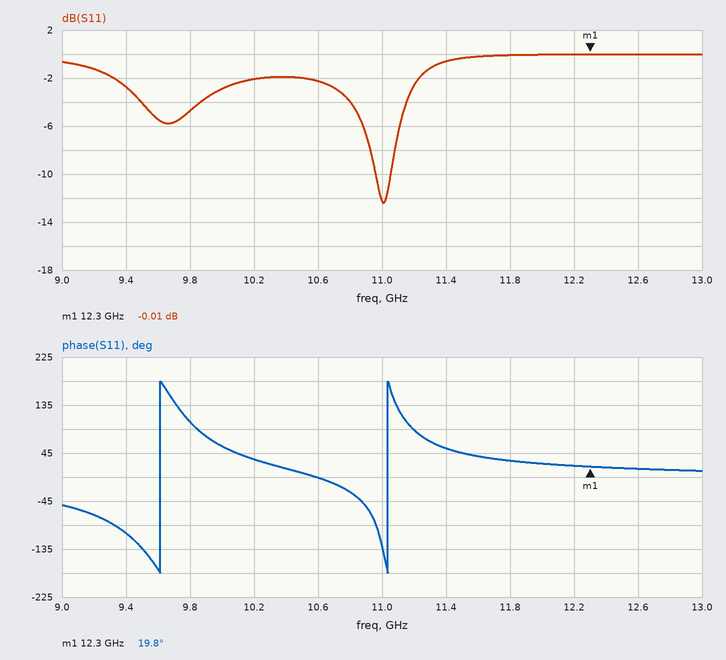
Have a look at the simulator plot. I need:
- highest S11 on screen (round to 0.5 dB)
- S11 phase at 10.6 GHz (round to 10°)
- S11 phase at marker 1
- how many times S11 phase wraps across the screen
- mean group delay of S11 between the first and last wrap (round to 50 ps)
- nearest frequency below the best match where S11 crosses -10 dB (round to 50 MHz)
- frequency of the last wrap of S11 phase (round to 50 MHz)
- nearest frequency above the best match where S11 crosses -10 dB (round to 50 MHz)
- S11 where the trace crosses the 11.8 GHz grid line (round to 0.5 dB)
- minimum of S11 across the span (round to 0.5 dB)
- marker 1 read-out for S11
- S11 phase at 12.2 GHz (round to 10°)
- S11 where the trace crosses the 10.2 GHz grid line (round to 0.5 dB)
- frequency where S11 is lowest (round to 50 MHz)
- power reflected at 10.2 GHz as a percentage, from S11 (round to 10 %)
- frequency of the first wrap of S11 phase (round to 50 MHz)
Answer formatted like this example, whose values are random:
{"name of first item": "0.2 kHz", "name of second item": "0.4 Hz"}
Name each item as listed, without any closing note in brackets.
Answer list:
{"highest S11 on screen": "0.0 dB", "S11 phase at 10.6 GHz": "0°", "S11 phase at marker 1": "19.8°", "how many times S11 phase wraps across the screen": "2", "mean group delay of S11 between the first and last wrap": "700 ps", "nearest frequency below the best match where S11 crosses -10 dB": "10.95 GHz", "frequency of the last wrap of S11 phase": "11.05 GHz", "nearest frequency above the best match where S11 crosses -10 dB": "11.05 GHz", "S11 where the trace crosses the 11.8 GHz grid line": "0.0 dB", "minimum of S11 across the span": "-12.5 dB", "marker 1 read-out for S11": "-0.01 dB", "S11 phase at 12.2 GHz": "20°", "S11 where the trace crosses the 10.2 GHz grid line": "-2.0 dB", "frequency where S11 is lowest": "11.00 GHz", "power reflected at 10.2 GHz as a percentage, from S11": "60 %", "frequency of the first wrap of S11 phase": "9.60 GHz"}
